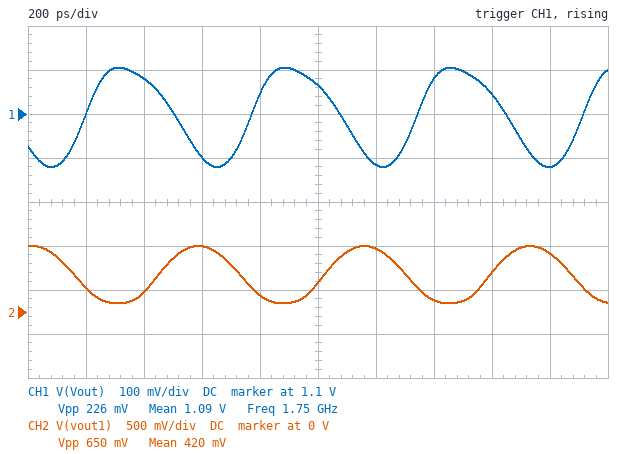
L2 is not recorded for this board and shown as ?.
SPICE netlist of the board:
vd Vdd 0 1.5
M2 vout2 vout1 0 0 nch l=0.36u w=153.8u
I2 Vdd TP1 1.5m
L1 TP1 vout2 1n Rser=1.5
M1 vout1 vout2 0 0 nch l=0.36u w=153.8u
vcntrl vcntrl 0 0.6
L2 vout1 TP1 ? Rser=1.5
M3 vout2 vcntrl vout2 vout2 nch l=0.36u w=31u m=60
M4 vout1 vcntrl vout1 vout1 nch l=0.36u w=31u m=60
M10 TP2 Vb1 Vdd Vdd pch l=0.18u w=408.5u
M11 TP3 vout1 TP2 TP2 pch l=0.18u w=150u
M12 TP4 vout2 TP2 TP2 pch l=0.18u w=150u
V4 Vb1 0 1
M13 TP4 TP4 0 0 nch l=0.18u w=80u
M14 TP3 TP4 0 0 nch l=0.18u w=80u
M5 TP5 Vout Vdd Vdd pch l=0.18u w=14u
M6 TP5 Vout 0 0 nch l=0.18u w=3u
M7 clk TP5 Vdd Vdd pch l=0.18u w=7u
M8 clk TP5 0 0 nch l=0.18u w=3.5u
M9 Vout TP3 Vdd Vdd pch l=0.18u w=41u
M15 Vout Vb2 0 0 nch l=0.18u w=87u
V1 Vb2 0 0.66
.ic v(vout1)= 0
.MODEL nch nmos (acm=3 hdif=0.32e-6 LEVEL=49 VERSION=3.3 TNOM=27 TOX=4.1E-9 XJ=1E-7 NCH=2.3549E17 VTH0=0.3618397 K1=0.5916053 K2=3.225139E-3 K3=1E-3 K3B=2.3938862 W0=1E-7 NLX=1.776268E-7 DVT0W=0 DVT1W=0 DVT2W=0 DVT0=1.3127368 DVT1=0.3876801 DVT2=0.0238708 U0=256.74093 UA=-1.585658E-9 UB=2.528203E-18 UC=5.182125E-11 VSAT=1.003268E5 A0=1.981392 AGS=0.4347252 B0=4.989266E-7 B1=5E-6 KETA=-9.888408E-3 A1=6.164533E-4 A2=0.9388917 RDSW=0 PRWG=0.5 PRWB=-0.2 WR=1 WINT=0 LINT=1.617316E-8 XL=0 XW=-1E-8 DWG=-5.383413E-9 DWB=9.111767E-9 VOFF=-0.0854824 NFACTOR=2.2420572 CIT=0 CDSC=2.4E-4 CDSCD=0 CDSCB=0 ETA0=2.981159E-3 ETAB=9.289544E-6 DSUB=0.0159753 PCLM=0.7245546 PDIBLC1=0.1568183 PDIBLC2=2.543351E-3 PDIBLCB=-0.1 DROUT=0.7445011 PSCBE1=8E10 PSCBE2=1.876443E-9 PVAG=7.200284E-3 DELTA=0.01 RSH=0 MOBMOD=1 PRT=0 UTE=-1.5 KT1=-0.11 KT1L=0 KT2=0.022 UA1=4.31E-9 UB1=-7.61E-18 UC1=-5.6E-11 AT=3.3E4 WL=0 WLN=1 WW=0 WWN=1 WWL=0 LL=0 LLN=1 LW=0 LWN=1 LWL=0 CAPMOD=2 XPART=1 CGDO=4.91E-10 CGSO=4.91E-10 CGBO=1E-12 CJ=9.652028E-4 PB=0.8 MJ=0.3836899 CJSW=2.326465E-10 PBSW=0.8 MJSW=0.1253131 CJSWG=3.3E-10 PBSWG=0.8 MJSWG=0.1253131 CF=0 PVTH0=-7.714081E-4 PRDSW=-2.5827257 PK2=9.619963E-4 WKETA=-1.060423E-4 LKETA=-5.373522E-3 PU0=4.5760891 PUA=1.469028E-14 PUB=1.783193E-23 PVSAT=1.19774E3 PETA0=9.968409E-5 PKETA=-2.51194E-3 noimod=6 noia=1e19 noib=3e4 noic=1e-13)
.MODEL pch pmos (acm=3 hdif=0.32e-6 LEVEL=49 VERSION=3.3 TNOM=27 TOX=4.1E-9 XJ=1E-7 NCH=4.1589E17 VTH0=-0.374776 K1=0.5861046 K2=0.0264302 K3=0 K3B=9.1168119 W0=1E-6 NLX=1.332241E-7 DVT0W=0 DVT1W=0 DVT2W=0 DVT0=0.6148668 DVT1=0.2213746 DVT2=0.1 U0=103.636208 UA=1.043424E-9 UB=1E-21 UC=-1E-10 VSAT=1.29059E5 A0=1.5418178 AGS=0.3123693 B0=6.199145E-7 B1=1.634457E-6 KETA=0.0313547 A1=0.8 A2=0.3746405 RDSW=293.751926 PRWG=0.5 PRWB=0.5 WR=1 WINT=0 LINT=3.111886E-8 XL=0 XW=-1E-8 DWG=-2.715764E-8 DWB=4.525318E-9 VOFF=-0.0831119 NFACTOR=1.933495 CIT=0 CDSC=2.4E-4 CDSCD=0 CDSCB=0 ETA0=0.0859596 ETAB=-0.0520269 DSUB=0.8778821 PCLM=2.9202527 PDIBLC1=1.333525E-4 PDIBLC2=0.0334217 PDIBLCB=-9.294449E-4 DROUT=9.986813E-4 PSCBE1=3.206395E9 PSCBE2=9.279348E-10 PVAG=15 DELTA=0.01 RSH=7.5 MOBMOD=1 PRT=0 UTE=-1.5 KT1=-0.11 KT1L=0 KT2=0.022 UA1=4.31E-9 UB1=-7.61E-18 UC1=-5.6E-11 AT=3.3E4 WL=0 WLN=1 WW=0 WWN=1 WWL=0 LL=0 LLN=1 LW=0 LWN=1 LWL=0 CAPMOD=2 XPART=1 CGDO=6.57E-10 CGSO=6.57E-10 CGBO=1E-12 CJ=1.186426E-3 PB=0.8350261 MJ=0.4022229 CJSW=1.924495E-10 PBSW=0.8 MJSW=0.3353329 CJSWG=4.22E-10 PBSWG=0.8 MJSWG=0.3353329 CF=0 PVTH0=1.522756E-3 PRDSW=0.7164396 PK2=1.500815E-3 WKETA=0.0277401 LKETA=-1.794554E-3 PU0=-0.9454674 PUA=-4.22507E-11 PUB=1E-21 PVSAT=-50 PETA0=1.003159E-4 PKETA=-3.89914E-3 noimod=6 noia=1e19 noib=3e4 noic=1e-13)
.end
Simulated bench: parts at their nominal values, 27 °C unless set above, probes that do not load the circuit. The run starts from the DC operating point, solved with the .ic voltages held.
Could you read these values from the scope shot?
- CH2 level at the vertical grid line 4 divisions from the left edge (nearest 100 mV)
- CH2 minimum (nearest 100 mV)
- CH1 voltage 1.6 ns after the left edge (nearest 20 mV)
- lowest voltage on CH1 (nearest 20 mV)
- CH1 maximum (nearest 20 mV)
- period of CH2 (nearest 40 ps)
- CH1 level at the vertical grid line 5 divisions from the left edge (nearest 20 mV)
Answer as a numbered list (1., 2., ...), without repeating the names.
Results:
1. 200 mV
2. 100 mV
3. 1.14 V
4. 980 mV
5. 1.20 V
6. 560 ps
7. 1.16 V
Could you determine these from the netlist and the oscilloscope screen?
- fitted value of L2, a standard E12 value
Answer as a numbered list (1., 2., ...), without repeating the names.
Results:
1. 2.7 nH
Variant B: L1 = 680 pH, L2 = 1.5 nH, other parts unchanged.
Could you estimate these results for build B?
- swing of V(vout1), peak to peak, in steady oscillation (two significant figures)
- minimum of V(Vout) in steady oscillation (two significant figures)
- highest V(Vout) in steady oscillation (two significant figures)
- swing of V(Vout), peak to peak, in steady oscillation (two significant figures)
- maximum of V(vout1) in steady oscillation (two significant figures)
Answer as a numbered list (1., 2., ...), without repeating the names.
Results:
1. 390 mV
2. 970 mV
3. 1.1 V
4. 150 mV
5. 690 mV
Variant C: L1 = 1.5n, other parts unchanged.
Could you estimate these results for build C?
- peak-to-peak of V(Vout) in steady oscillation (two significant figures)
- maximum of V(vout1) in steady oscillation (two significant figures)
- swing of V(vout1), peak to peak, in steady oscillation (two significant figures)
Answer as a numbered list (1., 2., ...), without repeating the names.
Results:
1. 240 mV
2. 780 mV
3. 710 mV
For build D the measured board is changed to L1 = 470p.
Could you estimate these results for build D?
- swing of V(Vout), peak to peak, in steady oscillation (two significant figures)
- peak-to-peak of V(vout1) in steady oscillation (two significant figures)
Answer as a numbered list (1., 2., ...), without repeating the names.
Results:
1. 210 mV
2. 590 mV
